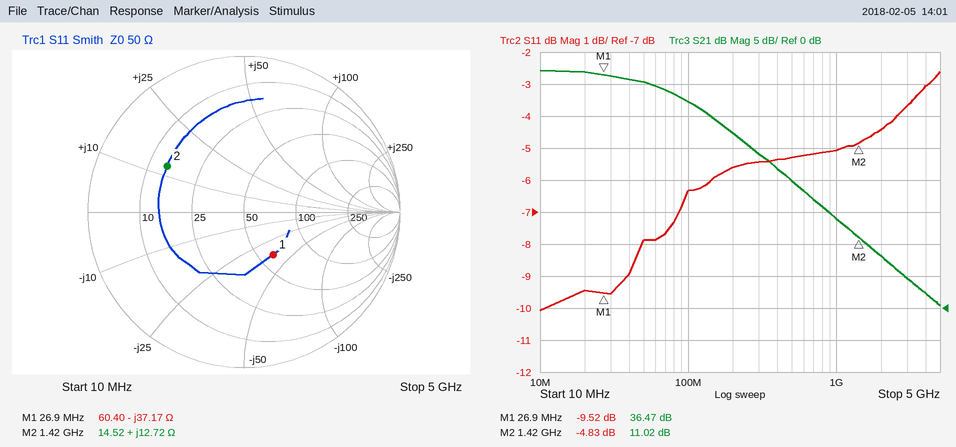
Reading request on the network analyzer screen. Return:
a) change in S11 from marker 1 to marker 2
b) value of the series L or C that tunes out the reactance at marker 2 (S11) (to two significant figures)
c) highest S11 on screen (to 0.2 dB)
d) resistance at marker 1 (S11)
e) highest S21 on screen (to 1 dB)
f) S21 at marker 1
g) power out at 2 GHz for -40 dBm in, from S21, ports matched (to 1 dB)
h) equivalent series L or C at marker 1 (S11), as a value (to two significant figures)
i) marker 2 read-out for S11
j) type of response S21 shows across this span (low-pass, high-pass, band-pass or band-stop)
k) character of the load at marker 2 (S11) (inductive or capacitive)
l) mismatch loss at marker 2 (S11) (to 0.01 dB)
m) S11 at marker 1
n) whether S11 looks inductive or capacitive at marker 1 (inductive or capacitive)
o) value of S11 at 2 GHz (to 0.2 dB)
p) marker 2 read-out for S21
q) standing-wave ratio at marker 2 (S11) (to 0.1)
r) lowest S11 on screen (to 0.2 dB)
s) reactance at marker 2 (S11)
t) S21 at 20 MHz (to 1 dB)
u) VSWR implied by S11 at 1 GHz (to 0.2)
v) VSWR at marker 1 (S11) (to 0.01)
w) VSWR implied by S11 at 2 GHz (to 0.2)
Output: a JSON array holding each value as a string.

["4.69 dB", "8.8 pF", "-2.6 dB", "60.40 Ω", "37 dB", "36.47 dB", "-32 dBm", "160 pF", "-4.83 dB", "low-pass", "inductive", "1.73 dB", "-9.52 dB", "capacitive", "-4.4 dB", "11.02 dB", "3.7", "-10.0 dB", "+12.72 Ω", "37 dB", "3.6", "1.99", "4.0"]
